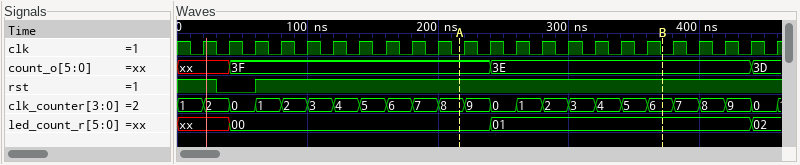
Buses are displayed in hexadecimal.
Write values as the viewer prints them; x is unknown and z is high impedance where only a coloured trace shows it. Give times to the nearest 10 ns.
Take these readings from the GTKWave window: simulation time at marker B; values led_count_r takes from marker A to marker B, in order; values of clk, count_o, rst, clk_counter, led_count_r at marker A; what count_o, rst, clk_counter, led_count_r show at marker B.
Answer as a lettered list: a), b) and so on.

a) 370 ns
b) 00, 01
c) clk=0, count_o=3F, rst=1, clk_counter=8, led_count_r=00
d) count_o=3E, rst=1, clk_counter=6, led_count_r=01
